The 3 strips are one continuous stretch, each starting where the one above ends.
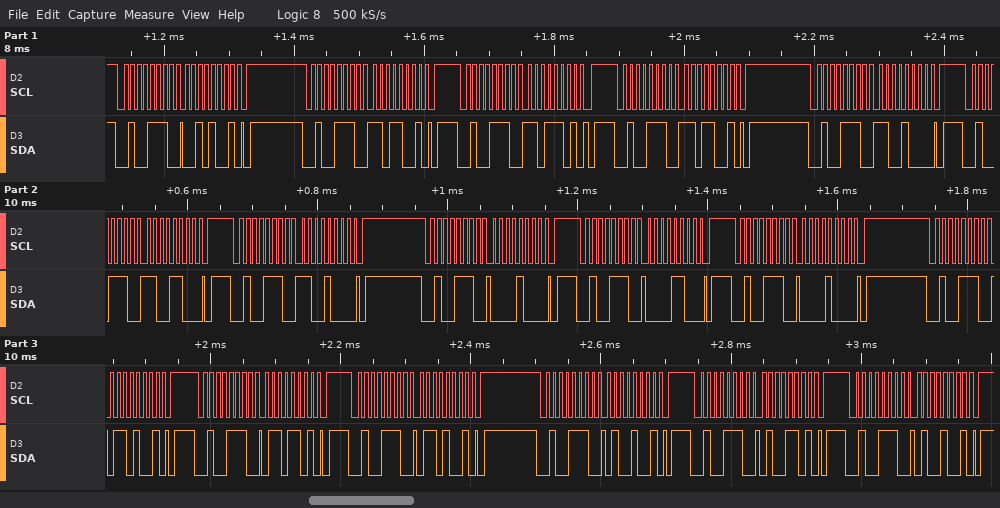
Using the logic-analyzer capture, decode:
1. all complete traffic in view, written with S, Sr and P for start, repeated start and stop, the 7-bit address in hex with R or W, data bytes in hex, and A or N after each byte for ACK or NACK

S 27W A 29 A P S 27W A D9 A P S 27W A DD A P S 27W A D9 A P S 27W A C8 A P S 27W A CC A P S 27W A C8 A P S 27W A 08 A P S 27W A 0C A P S 27W A 08 A P S 27W A 69 A P S 27W A 6D A P S 27W A 69 A P S 27W A 49 A P S 27W A 4D A P S 27W A 49 A P
